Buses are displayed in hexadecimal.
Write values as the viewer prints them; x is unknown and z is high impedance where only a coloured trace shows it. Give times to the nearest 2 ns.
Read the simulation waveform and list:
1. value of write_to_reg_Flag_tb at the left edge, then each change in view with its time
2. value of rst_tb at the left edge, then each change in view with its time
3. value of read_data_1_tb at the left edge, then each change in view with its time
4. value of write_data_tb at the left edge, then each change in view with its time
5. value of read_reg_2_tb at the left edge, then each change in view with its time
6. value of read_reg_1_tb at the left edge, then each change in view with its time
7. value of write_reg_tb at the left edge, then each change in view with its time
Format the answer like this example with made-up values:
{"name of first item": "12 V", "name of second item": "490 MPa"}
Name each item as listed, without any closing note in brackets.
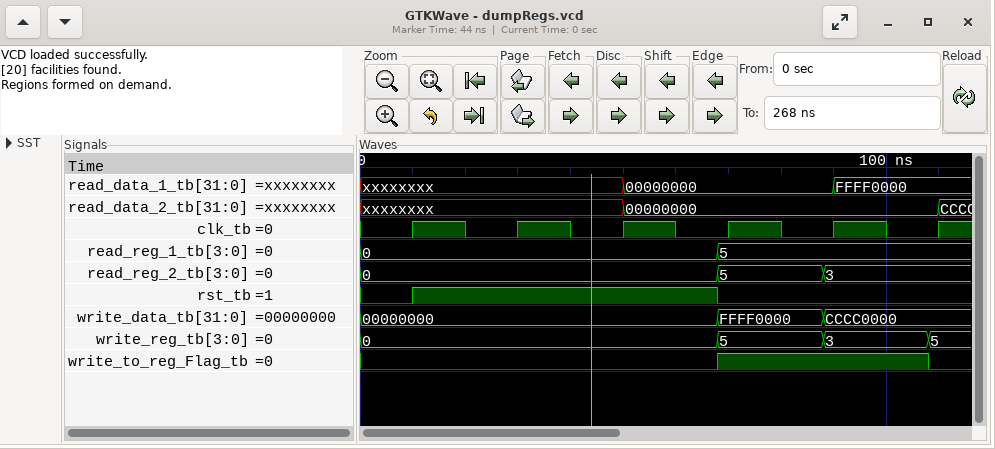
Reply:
{"value of write_to_reg_Flag_tb at the left edge, then each change in view with its time": "0, 1 at 68 ns, 0 at 108 ns", "value of rst_tb at the left edge, then each change in view with its time": "0, 1 at 10 ns, 0 at 68 ns", "value of read_data_1_tb at the left edge, then each change in view with its time": "xxxxxxxx, 00000000 at 50 ns, FFFF0000 at 90 ns", "value of write_data_tb at the left edge, then each change in view with its time": "00000000, FFFF0000 at 68 ns, CCCC0000 at 88 ns", "value of read_reg_2_tb at the left edge, then each change in view with its time": "0, 5 at 68 ns, 3 at 88 ns", "value of read_reg_1_tb at the left edge, then each change in view with its time": "0, 5 at 68 ns", "value of write_reg_tb at the left edge, then each change in view with its time": "0, 5 at 68 ns, 3 at 88 ns, 5 at 108 ns"}
